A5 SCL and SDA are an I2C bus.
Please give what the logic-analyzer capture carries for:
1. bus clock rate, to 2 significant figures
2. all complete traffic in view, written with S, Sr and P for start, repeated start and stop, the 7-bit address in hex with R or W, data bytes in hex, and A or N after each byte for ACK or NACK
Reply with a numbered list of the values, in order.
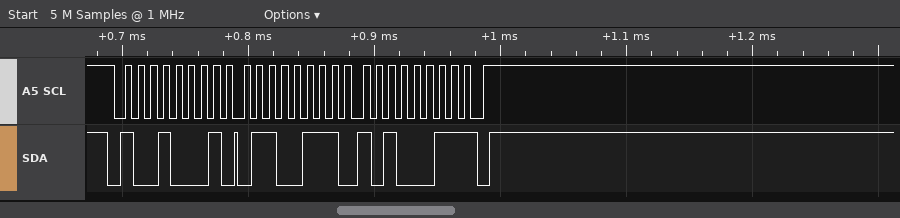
1. 100 kHz
2. S 48R A 67 A A3 N P
